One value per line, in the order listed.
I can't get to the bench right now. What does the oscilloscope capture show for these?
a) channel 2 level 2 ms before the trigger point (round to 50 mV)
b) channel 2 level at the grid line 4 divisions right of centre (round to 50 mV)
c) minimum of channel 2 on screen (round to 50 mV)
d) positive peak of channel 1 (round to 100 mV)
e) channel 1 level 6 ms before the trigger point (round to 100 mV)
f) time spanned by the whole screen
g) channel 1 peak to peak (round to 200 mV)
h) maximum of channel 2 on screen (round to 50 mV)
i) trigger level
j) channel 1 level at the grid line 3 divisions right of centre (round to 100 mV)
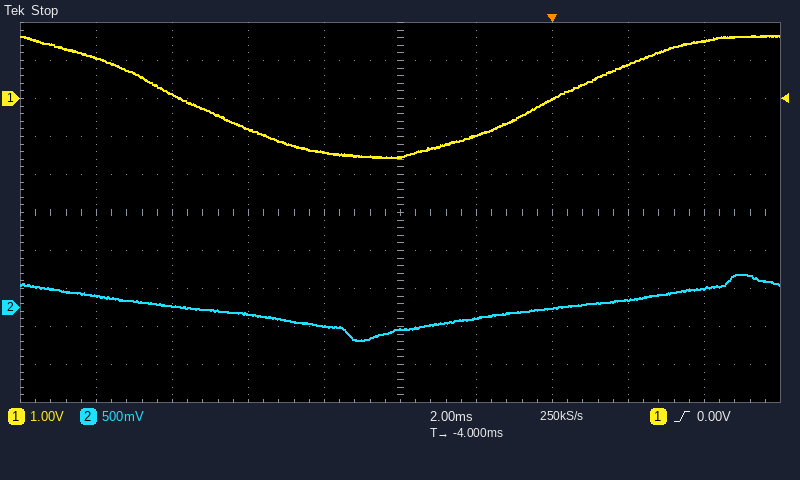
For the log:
-150 mV
250 mV
-450 mV
1.7 V
-1.4 V
20 ms
3.2 V
450 mV
0.00 V
900 mV
